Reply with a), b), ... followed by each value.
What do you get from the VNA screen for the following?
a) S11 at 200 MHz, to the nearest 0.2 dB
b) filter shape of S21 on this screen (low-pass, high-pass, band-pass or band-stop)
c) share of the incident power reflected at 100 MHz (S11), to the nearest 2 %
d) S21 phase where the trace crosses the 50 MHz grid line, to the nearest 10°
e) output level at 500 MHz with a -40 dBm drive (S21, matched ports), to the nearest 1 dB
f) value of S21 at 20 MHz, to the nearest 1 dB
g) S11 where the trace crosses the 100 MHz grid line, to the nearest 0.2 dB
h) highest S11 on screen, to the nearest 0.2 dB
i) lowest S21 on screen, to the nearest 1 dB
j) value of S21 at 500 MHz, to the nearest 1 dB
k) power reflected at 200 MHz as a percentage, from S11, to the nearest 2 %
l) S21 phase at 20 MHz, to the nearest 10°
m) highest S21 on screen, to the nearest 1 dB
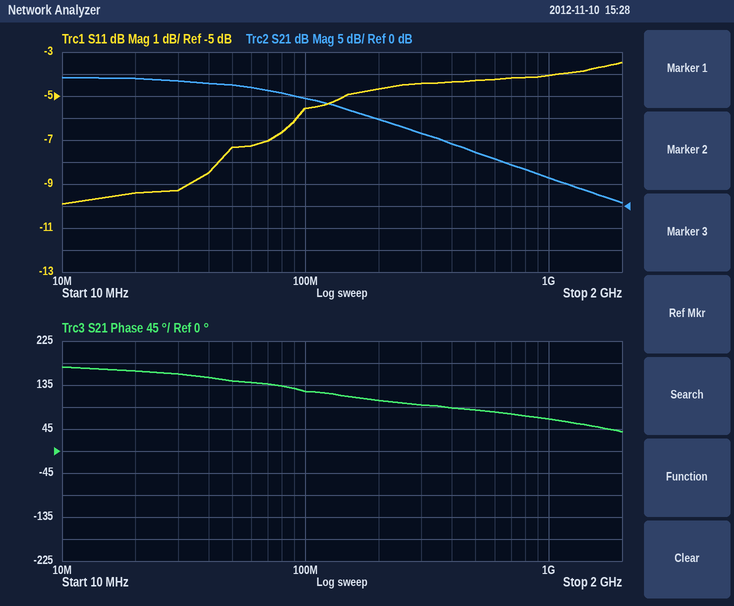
a) -4.6 dB
b) low-pass
c) 28 %
d) 140°
e) -28 dBm
f) 29 dB
g) -5.6 dB
h) -3.4 dB
i) 1 dB
j) 12 dB
k) 34 %
l) 160°
m) 29 dB
